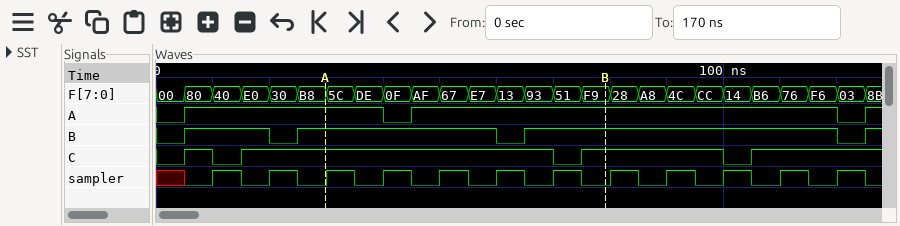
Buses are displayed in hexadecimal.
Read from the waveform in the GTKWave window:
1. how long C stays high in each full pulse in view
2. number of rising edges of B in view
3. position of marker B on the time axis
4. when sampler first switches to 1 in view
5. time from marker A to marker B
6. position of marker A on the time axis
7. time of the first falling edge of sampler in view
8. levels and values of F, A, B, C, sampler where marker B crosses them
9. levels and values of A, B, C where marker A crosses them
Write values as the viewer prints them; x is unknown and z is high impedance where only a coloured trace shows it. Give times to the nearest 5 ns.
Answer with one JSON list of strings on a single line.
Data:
["5 ns, 55 ns, 25 ns", "4", "80 ns", "10 ns", "50 ns", "30 ns", "15 ns", "F=F9, A=1, B=1, C=1, sampler=0", "A=1, B=1, C=1"]
